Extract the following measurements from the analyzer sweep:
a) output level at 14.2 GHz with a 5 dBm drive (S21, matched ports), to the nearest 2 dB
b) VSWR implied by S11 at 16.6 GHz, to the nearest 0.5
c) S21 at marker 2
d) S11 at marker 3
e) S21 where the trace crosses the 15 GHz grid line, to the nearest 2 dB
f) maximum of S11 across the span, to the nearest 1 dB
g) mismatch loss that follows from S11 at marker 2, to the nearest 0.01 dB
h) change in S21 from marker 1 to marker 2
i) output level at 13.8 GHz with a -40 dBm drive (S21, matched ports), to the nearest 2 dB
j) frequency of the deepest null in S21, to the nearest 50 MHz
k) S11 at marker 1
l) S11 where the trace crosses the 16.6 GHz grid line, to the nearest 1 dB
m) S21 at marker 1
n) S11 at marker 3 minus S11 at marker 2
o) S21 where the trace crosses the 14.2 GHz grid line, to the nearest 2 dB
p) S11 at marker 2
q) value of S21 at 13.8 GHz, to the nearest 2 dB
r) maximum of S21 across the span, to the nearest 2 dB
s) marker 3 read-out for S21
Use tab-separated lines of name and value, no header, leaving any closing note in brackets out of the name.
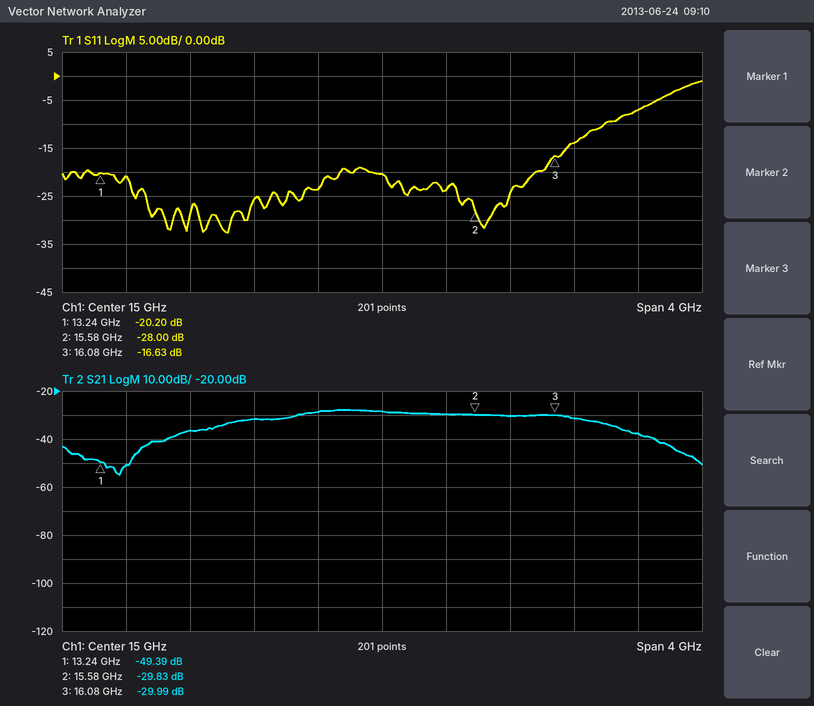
output level at 14.2 GHz with a 5 dBm drive (S21, matched ports), to the nearest 2 dB	-26 dBm
VSWR implied by S11 at 16.6 GHz, to the nearest 0.5	2.5
S21 at marker 2	-29.83 dB
S11 at marker 3	-16.63 dB
S21 where the trace crosses the 15 GHz grid line, to the nearest 2 dB	-28 dB
maximum of S11 across the span, to the nearest 1 dB	-1 dB
mismatch loss that follows from S11 at marker 2, to the nearest 0.01 dB	0.01 dB
change in S21 from marker 1 to marker 2	19.56 dB
output level at 13.8 GHz with a -40 dBm drive (S21, matched ports), to the nearest 2 dB	-76 dBm
frequency of the deepest null in S21, to the nearest 50 MHz	13.35 GHz
S11 at marker 1	-20.20 dB
S11 where the trace crosses the 16.6 GHz grid line, to the nearest 1 dB	-7 dB
S21 at marker 1	-49.39 dB
S11 at marker 3 minus S11 at marker 2	11.37 dB
S21 where the trace crosses the 14.2 GHz grid line, to the nearest 2 dB	-32 dB
S11 at marker 2	-28.00 dB
value of S21 at 13.8 GHz, to the nearest 2 dB	-36 dB
maximum of S21 across the span, to the nearest 2 dB	-28 dB
marker 3 read-out for S21	-29.99 dB
